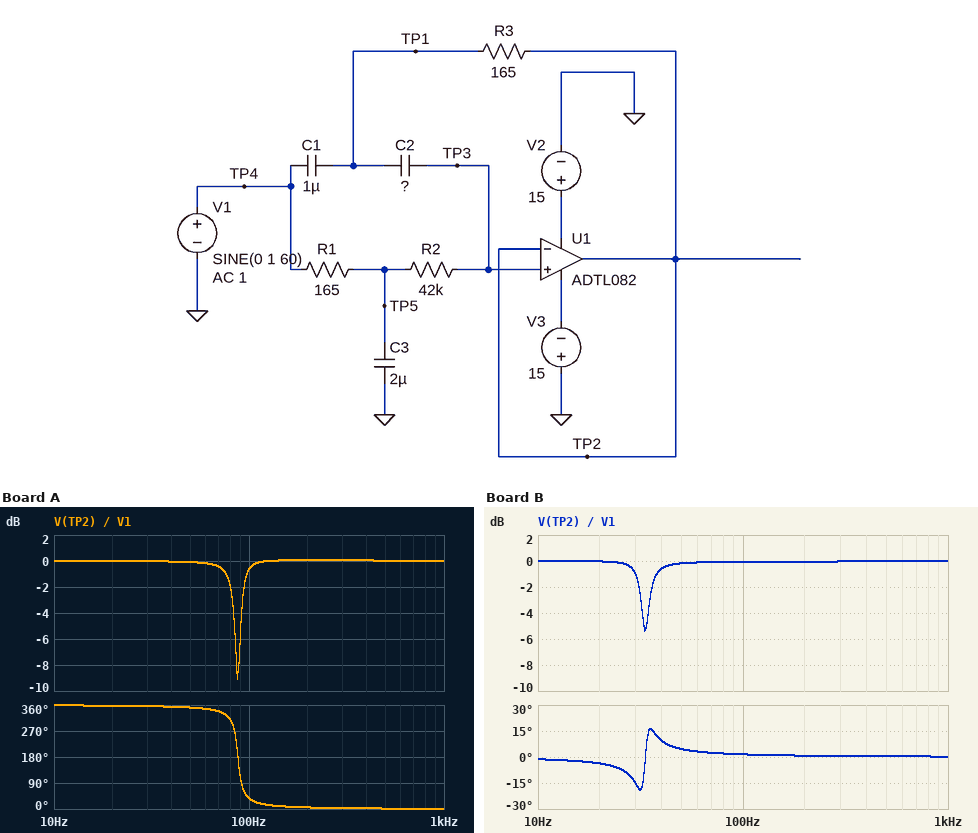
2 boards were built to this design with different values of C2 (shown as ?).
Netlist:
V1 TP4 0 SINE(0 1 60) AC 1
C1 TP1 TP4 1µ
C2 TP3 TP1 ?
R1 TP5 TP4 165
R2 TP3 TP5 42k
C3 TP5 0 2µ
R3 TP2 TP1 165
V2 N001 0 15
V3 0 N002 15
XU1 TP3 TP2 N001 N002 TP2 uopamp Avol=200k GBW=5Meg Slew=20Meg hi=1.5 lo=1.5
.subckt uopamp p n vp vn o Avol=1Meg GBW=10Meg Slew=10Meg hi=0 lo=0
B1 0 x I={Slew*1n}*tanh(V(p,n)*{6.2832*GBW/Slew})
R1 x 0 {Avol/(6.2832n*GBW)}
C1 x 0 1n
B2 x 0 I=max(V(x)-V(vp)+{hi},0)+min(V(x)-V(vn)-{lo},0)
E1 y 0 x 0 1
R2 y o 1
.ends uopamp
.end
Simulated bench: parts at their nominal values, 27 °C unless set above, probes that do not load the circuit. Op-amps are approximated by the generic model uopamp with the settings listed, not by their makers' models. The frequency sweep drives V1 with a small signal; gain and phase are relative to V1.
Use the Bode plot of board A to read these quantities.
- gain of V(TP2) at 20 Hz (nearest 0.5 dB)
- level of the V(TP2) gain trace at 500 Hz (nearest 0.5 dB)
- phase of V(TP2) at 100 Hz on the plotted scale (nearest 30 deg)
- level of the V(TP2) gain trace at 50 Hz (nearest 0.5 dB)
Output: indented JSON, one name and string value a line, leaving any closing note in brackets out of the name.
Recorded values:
{
  "gain of V(TP2) at 20 Hz": "0 dB",
  "level of the V(TP2) gain trace at 500 Hz": "0 dB",
  "phase of V(TP2) at 100 Hz on the plotted scale": "30 deg",
  "level of the V(TP2) gain trace at 50 Hz": "0 dB"
}
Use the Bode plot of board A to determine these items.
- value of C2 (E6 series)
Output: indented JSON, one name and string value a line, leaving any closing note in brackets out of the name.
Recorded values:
{
  "value of C2": "470 nF"
}
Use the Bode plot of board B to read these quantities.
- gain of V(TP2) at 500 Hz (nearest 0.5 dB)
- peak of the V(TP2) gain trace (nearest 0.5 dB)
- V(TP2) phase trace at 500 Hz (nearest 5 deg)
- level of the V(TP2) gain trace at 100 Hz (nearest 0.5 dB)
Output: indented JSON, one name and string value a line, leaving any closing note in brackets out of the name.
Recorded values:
{
  "gain of V(TP2) at 500 Hz": "0 dB",
  "peak of the V(TP2) gain trace": "0 dB",
  "V(TP2) phase trace at 500 Hz": "0 deg",
  "level of the V(TP2) gain trace at 100 Hz": "0 dB"
}
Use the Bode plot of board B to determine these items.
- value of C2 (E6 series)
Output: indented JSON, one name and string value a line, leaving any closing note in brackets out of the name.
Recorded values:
{
  "value of C2": "3.3 µF"
}
